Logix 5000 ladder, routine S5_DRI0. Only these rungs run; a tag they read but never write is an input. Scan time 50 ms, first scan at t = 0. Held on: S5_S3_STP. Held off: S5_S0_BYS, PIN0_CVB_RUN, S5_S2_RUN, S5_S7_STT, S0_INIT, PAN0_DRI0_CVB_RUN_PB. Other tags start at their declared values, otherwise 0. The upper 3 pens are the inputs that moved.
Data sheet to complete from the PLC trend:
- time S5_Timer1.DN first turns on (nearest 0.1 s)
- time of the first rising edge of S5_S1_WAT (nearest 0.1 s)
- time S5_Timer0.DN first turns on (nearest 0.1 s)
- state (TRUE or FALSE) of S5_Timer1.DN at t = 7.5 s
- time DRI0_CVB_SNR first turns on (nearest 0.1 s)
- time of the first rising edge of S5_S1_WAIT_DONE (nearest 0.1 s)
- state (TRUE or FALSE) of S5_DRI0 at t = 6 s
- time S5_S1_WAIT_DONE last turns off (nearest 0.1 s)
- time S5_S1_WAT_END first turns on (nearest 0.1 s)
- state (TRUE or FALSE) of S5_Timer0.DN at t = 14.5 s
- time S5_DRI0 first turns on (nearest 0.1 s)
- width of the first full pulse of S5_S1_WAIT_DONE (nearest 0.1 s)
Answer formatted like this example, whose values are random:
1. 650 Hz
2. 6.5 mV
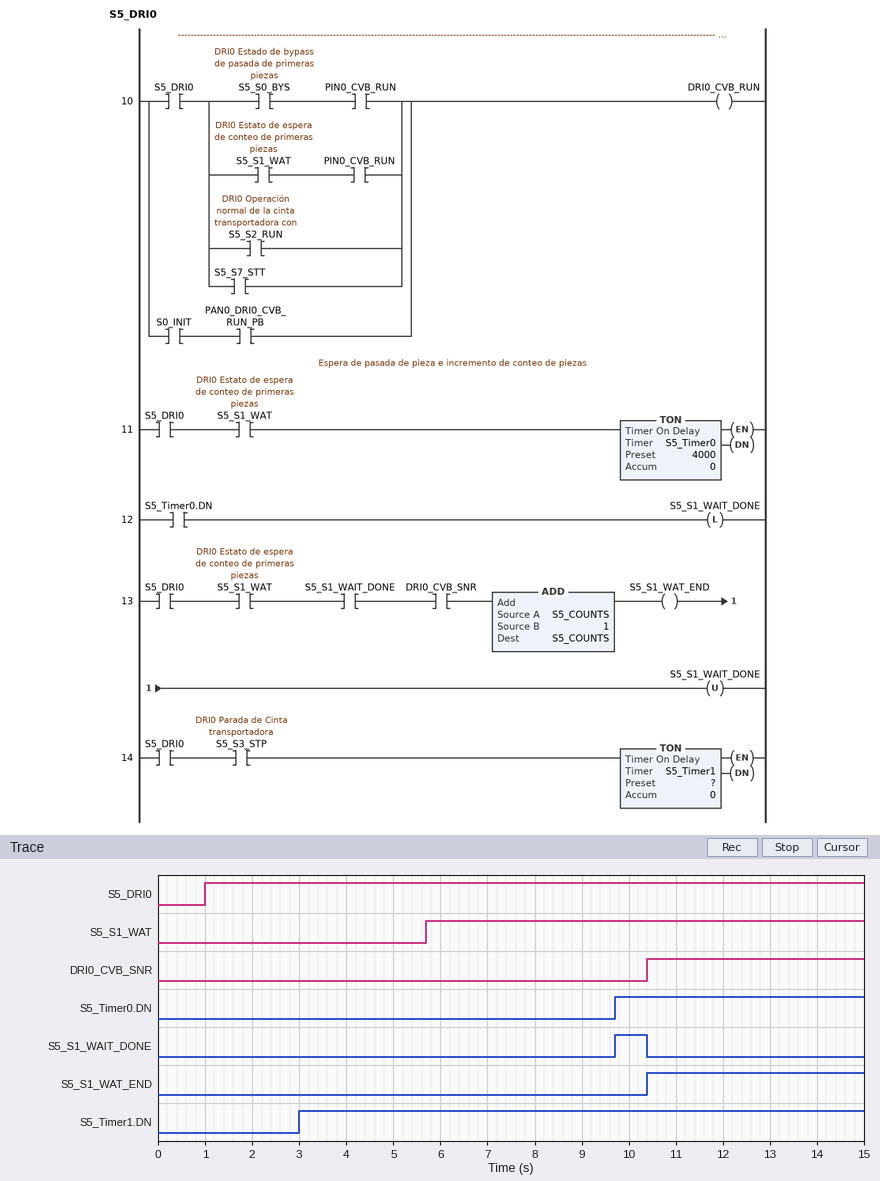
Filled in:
1. 3.0 s
2. 5.7 s
3. 9.7 s
4. TRUE
5. 10.4 s
6. 9.7 s
7. TRUE
8. 10.4 s
9. 10.4 s
10. TRUE
11. 1.0 s
12. 0.7 s
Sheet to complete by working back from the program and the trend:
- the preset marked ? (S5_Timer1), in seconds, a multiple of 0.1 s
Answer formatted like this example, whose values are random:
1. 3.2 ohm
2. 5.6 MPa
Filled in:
1. 2.0 s
